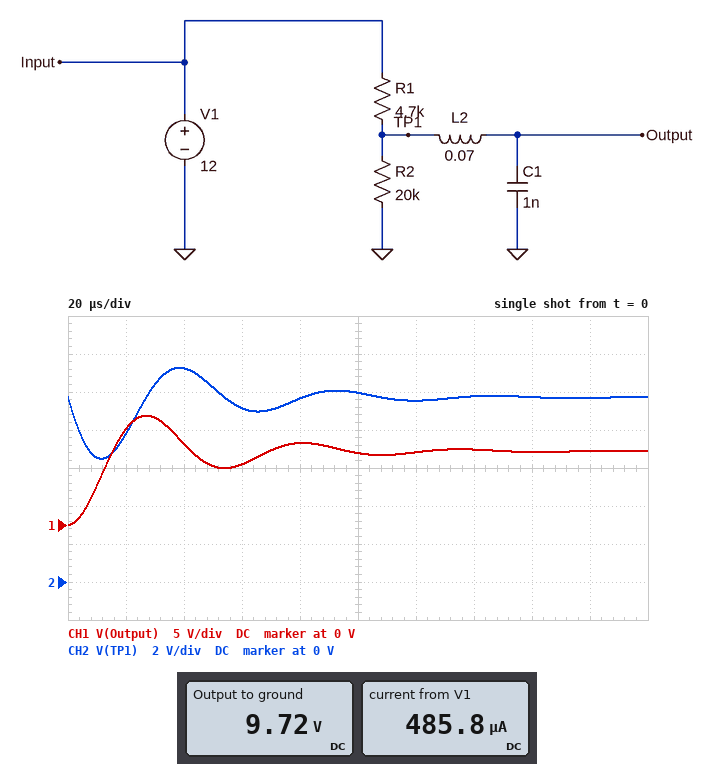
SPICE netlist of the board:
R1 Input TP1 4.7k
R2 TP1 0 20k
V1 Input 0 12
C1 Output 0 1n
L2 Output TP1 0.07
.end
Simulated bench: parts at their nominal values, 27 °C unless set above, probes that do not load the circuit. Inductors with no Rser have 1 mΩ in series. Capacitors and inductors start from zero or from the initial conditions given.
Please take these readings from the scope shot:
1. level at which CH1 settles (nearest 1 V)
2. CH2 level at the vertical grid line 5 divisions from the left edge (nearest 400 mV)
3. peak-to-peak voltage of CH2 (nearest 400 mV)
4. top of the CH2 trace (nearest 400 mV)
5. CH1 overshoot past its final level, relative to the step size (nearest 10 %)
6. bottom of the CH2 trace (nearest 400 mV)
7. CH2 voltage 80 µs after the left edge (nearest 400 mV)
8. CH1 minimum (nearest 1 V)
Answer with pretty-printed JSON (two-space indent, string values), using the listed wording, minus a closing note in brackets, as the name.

{
  "level at which CH1 settles": "10 V",
  "CH2 level at the vertical grid line 5 divisions from the left edge": "10.0 V",
  "peak-to-peak voltage of CH2": "4.8 V",
  "top of the CH2 trace": "11.2 V",
  "CH1 overshoot past its final level, relative to the step size": "50 %",
  "bottom of the CH2 trace": "6.4 V",
  "CH2 voltage 80 µs after the left edge": "9.6 V",
  "CH1 minimum": "0 V"
}
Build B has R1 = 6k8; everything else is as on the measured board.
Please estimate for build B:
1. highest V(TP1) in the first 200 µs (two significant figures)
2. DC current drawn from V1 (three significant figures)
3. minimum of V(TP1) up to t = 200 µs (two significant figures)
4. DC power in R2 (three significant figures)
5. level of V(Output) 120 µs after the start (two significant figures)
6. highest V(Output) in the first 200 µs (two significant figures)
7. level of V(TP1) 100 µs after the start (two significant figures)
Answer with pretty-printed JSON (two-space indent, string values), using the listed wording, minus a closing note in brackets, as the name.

{
  "highest V(TP1) in the first 200 µs": "10 V",
  "DC current drawn from V1": "448 µA",
  "minimum of V(TP1) up to t = 200 µs": "5.3 V",
  "DC power in R2": "4.01 mW",
  "level of V(Output) 120 µs after the start": "8.9 V",
  "highest V(Output) in the first 200 µs": "12 V",
  "level of V(TP1) 100 µs after the start": "9.1 V"
}
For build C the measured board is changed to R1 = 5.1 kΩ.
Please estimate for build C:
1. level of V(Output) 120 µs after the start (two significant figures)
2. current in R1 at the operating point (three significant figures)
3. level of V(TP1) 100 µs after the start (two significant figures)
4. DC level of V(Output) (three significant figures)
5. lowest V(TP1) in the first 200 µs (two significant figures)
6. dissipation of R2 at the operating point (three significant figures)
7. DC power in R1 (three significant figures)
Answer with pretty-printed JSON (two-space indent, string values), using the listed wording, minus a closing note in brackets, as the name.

{
  "level of V(Output) 120 µs after the start": "9.4 V",
  "current in R1 at the operating point": "478 µA",
  "level of V(TP1) 100 µs after the start": "9.8 V",
  "DC level of V(Output)": "9.56 V",
  "lowest V(TP1) in the first 200 µs": "6.2 V",
  "dissipation of R2 at the operating point": "4.57 mW",
  "DC power in R1": "1.17 mW"
}
